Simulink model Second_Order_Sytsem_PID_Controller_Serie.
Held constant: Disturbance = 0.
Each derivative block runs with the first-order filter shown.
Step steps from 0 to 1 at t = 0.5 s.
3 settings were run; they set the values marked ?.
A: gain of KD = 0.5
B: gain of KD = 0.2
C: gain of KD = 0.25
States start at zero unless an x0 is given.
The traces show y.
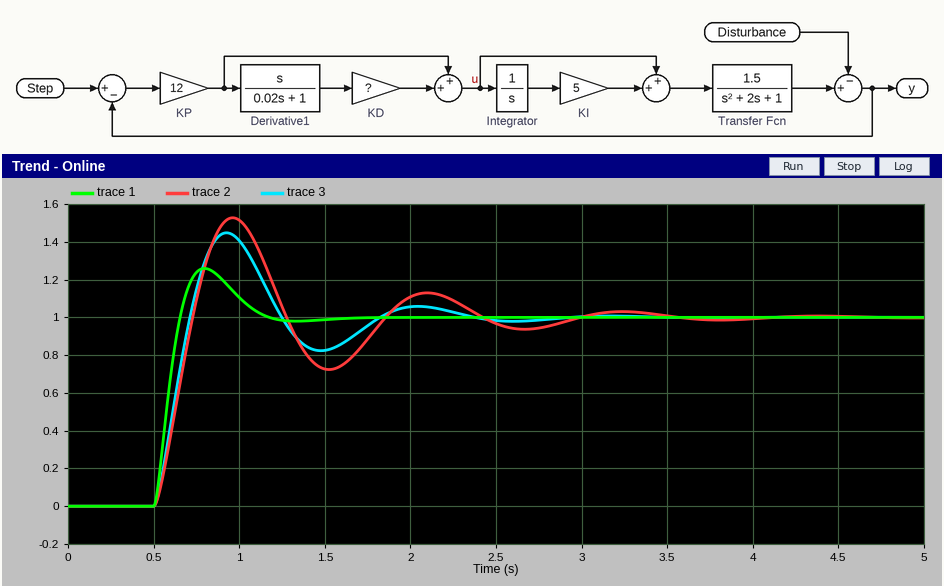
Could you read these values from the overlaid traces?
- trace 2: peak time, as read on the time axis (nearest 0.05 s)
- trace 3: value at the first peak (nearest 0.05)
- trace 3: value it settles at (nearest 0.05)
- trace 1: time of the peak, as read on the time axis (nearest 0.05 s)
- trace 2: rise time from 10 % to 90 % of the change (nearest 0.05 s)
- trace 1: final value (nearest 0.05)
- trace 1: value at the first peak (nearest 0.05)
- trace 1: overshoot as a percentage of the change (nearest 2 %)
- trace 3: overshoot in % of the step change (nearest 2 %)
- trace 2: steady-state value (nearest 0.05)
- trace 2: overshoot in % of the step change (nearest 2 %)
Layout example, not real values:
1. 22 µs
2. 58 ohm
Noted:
1. 0.95 s
2. 1.45
3. 1.00
4. 0.80 s
5. 0.15 s
6. 1.00
7. 1.25
8. 26 %
9. 44 %
10. 1.00
11. 52 %
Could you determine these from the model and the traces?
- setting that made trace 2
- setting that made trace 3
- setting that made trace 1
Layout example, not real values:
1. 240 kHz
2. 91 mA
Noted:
1. B
2. C
3. A
